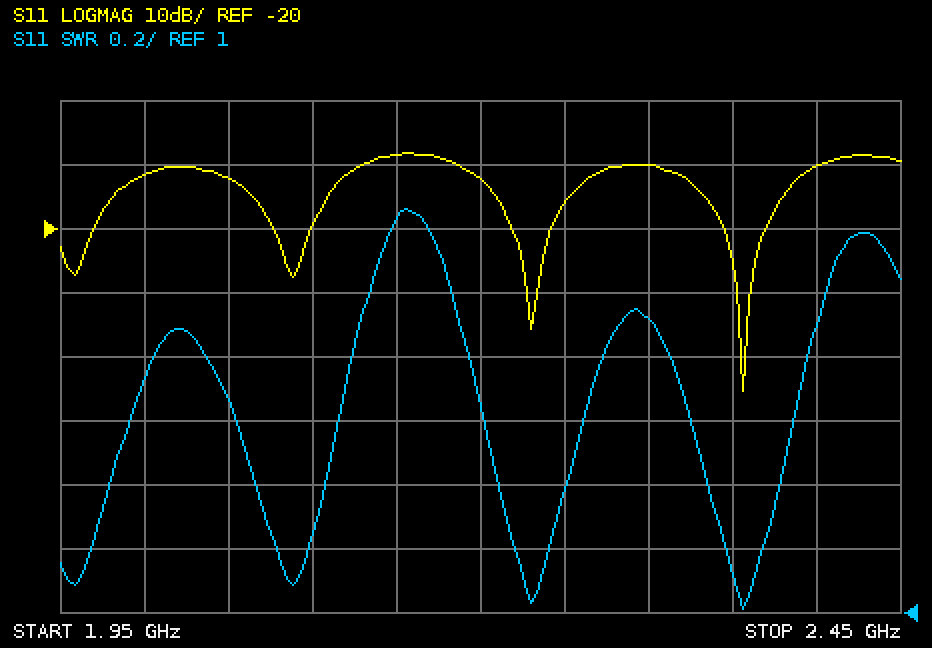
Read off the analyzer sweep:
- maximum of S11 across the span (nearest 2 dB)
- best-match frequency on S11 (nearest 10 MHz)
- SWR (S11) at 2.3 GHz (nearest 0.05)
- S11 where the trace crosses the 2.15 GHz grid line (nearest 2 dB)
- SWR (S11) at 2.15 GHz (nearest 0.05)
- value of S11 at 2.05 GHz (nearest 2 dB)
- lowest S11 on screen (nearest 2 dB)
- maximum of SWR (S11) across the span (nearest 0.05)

-8 dB
2.36 GHz
1.90
-8 dB
2.25
-12 dB
-46 dB
2.25
